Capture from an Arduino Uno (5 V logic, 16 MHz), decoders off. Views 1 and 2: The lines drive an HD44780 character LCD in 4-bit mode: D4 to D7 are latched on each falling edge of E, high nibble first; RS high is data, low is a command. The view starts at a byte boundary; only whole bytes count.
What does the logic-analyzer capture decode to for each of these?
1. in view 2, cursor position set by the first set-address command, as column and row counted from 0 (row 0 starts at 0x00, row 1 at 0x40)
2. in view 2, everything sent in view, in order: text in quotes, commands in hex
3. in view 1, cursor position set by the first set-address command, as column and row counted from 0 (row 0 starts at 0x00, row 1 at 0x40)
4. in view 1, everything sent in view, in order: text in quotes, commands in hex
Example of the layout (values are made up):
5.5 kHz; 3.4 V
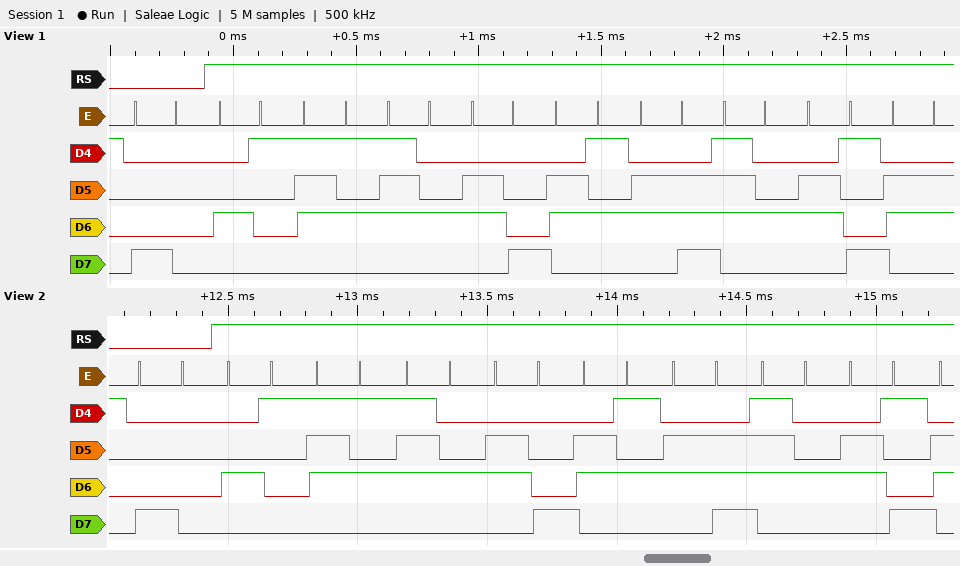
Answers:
column 0, row 0; 0x80 "Authenti"; column 0, row 0; 0x80 "Authentif"
